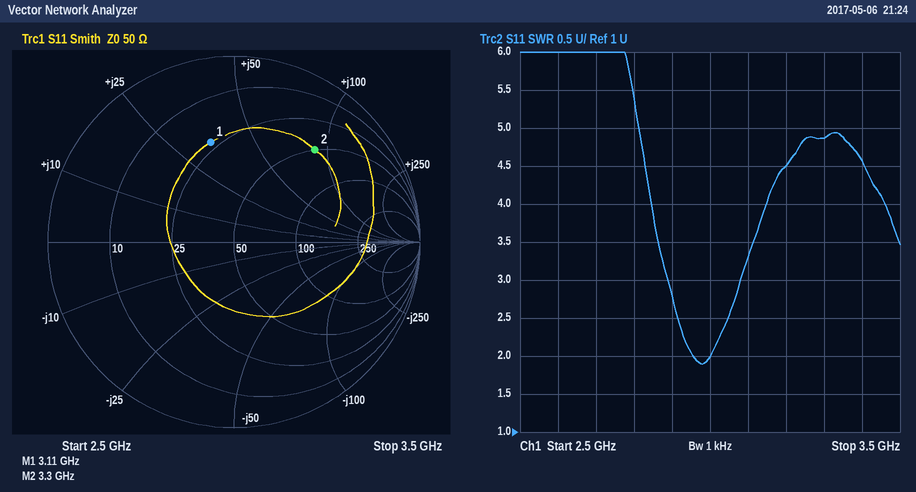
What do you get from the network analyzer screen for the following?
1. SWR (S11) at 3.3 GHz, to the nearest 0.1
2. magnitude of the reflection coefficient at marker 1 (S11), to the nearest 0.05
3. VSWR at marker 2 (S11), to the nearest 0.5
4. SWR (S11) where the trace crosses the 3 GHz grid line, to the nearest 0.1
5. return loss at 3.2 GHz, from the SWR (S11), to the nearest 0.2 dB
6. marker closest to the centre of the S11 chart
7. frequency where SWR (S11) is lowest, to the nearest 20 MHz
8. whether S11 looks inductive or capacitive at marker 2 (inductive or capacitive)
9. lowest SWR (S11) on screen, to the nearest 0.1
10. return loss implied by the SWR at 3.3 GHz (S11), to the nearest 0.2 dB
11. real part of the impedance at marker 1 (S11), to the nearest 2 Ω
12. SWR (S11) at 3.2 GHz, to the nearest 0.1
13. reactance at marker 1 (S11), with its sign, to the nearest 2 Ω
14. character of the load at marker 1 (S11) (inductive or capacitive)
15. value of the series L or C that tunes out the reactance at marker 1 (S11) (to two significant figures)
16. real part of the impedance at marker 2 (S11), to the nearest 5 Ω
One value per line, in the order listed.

4.9
0.55
5.0
2.0
4.0 dB
marker 1
2.98 GHz
inductive
1.9
3.6 dB
22 Ω
4.5
+34 Ω
inductive
1.5 pF
50 Ω
